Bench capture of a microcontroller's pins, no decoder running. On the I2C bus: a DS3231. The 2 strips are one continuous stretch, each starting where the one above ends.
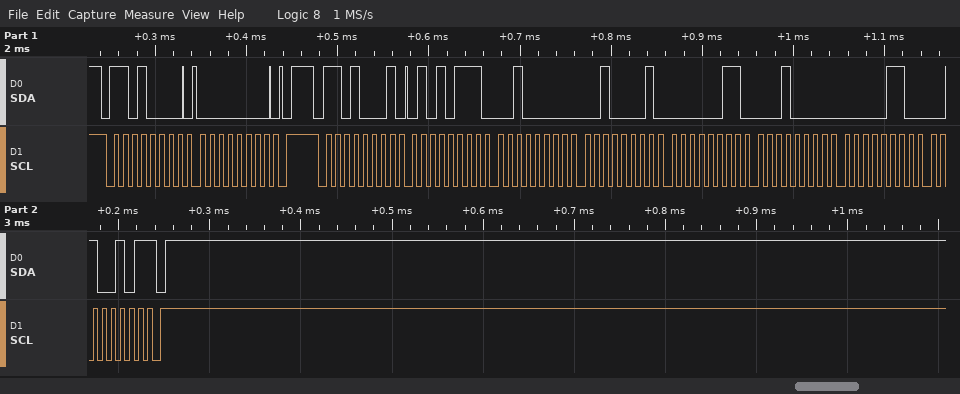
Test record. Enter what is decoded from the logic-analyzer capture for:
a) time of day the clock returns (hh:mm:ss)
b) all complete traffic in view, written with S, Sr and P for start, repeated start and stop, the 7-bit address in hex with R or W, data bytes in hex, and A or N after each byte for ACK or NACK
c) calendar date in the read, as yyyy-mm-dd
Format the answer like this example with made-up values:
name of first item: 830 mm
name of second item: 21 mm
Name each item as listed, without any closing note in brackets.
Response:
time of day the clock returns: 21:20:57
all complete traffic in view, written with S, Sr and P for start, repeated start and stop, the 7-bit address in hex with R or W, data bytes in hex, and A or N after each byte for ACK or NACK: S 68W A 00 A P S 68R A 57 A 20 A 21 A 03 A 10 A 06 A 25 N P
calendar date in the read, as yyyy-mm-dd: 2025-06-10
